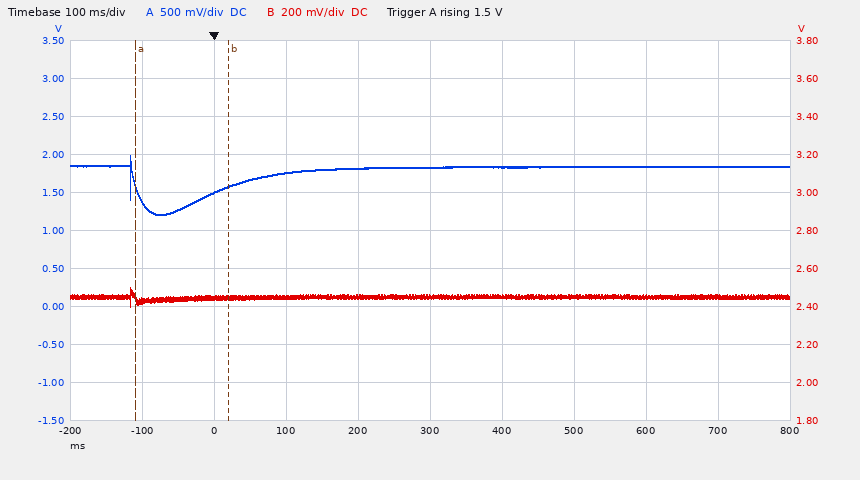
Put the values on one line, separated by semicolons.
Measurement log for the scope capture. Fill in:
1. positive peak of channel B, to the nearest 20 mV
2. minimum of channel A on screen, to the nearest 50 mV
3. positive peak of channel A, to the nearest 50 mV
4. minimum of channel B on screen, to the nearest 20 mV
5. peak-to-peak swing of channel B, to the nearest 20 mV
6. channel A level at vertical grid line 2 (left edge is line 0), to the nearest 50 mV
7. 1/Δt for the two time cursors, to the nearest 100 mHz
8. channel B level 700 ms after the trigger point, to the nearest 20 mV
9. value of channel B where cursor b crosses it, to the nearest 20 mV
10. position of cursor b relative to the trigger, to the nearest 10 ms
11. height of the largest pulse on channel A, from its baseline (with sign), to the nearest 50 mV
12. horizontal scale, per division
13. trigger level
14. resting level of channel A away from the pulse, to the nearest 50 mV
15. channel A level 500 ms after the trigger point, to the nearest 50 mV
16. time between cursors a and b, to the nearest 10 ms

2.50 V; 1.20 V; 2.00 V; 2.40 V; 100 mV; 1.50 V; 7.7 Hz; 2.46 V; 2.44 V; +20 ms; -650 mV; 100 ms; 1.5 V; 1.85 V; 1.85 V; 130 ms
